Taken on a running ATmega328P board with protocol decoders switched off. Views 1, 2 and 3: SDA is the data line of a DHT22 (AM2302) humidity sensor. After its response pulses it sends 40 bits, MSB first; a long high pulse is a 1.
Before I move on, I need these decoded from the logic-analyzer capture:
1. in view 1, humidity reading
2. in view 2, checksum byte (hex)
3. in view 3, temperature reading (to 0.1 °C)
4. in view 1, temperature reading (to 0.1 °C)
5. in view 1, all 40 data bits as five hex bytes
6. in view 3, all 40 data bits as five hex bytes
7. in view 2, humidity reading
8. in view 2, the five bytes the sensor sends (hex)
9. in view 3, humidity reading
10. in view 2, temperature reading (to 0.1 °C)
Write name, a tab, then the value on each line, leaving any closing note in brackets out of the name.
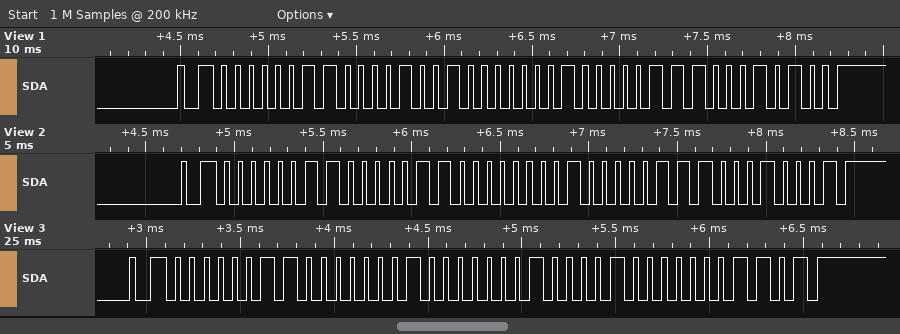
in view 1, humidity reading	77.7 %
in view 2, checksum byte	0x11
in view 3, temperature reading	26.4 °C
in view 1, temperature reading	26.3 °C
in view 1, all 40 data bits as five hex bytes	03 09 01 07 14
in view 3, all 40 data bits as five hex bytes	03 01 01 08 0D
in view 2, humidity reading	77.4 %
in view 2, the five bytes the sensor sends	03 06 01 07 11
in view 3, humidity reading	76.9 %
in view 2, temperature reading	26.3 °C
